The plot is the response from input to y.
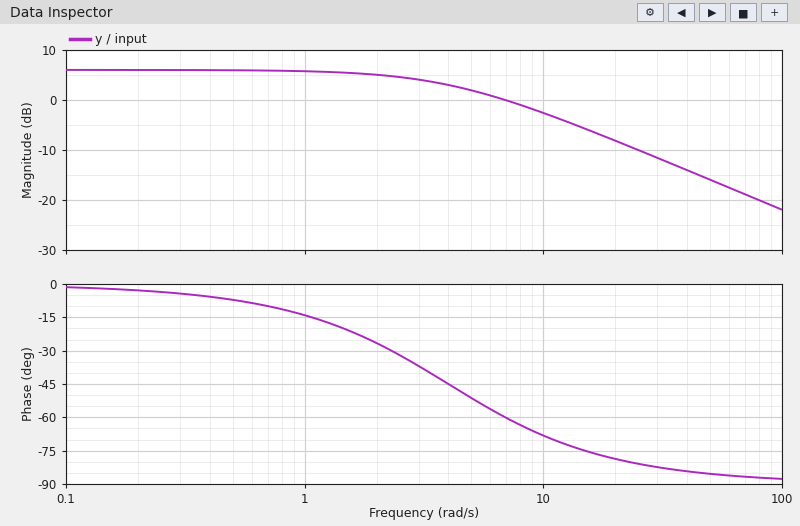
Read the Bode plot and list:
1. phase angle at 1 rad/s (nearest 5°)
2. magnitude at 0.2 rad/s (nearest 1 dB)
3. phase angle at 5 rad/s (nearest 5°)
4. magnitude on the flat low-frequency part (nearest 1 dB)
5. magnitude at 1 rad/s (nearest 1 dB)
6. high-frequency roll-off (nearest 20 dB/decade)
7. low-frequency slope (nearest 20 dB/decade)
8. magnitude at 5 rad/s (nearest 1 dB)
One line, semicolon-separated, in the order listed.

-15°; 6 dB; -50°; 6 dB; 6 dB; -20 dB/decade; 0 dB/decade; 2 dB
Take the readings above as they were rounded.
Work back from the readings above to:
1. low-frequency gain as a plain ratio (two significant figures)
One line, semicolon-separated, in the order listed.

2.0
